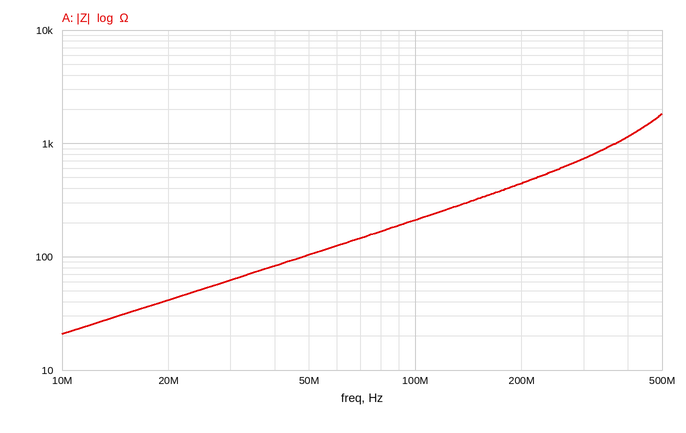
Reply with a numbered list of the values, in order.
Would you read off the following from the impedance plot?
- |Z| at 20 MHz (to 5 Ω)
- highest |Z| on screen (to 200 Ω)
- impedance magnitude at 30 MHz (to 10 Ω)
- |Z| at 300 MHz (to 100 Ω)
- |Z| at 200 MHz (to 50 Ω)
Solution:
1. 40 Ω
2. 1.8 kΩ
3. 60 Ω
4. 700 Ω
5. 450 Ω
